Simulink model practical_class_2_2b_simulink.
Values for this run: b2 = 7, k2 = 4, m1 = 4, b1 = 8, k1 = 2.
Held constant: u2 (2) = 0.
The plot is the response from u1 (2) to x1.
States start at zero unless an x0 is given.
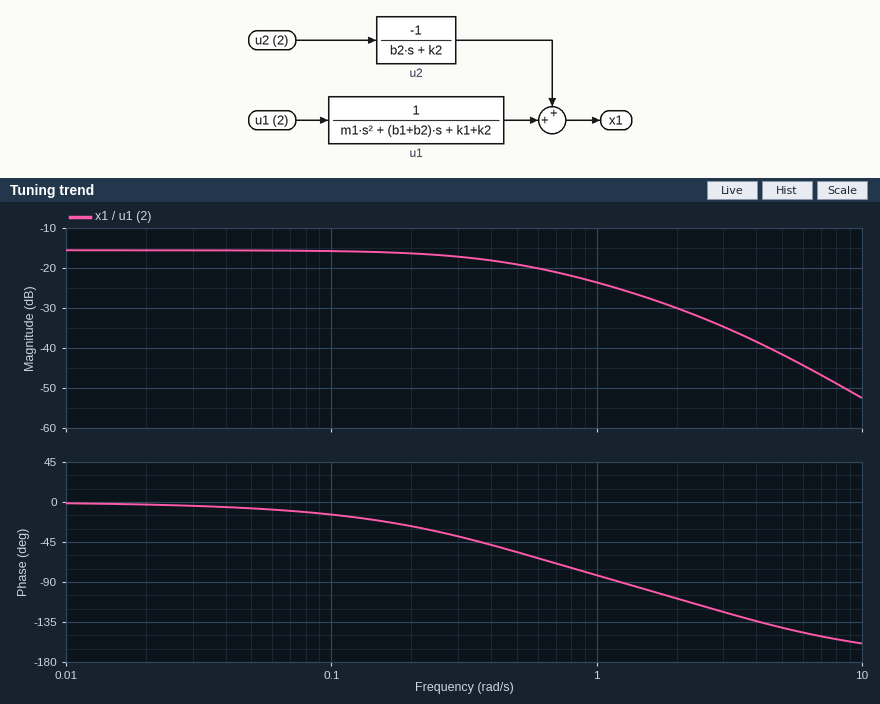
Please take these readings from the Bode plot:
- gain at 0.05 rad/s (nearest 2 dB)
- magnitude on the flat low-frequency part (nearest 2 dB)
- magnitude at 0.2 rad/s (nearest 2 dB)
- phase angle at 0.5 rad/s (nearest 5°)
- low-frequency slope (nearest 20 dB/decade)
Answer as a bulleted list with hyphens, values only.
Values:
- -16 dB
- -16 dB
- -16 dB
- -55°
- 0 dB/decade
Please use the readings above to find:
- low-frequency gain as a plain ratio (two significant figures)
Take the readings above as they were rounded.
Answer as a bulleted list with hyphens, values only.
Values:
- 0.16
